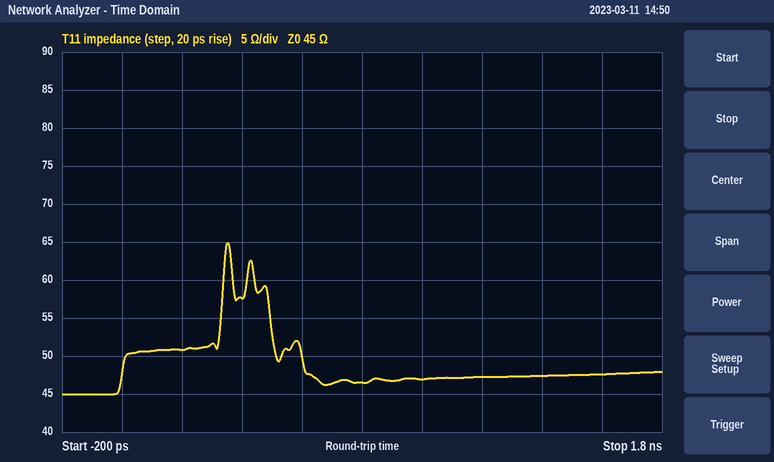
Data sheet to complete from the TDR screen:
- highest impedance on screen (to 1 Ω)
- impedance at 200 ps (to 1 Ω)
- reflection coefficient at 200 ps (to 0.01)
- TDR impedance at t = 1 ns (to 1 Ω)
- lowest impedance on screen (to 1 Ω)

65 Ω
51 Ω
+0.06
47 Ω
45 Ω
